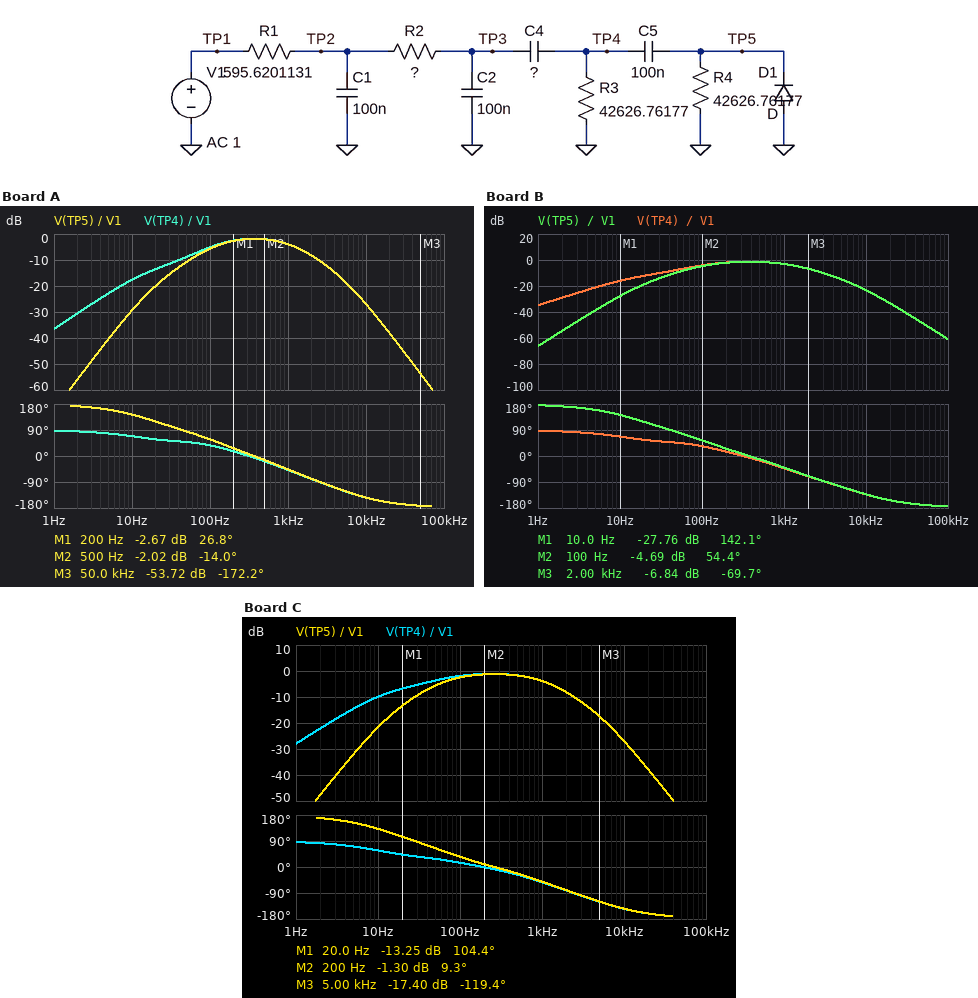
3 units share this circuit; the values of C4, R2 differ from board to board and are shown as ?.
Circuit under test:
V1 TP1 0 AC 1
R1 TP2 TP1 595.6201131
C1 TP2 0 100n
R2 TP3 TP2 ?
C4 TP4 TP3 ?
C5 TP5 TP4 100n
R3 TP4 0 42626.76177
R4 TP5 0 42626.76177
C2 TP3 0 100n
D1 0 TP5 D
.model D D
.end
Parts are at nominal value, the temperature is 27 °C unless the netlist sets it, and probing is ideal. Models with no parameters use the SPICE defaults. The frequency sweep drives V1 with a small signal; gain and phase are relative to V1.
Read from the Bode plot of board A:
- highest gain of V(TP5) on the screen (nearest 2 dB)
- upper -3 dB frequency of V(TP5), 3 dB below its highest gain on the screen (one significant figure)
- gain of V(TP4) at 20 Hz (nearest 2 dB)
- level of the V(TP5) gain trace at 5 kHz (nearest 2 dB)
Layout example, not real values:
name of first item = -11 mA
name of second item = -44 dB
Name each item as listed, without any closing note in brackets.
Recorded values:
highest gain of V(TP5) on the screen = -2 dB
upper -3 dB frequency of V(TP5), 3 dB below its highest gain on the screen = 1 kHz
gain of V(TP4) at 20 Hz = -14 dB
level of the V(TP5) gain trace at 5 kHz = -18 dB
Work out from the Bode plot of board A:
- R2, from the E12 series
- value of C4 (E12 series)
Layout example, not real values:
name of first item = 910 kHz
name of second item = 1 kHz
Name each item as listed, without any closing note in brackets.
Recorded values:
R2, from the E12 series = 820 Ω
value of C4 = 56 nF
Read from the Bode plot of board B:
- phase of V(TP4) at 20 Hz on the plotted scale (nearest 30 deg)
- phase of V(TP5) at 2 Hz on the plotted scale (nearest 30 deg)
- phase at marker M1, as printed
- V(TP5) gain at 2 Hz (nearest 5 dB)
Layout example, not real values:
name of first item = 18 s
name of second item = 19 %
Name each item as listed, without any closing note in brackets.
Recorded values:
phase of V(TP4) at 20 Hz on the plotted scale = 60 deg
phase of V(TP5) at 2 Hz on the plotted scale = 180 deg
phase at marker M1, as printed = 142.1 deg
V(TP5) gain at 2 Hz = -55 dB
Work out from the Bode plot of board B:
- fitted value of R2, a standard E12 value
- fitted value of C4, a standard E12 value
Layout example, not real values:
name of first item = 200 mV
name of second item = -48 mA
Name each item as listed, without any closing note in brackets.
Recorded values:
fitted value of R2, a standard E12 value = 470 Ω
fitted value of C4, a standard E12 value = 68 nF
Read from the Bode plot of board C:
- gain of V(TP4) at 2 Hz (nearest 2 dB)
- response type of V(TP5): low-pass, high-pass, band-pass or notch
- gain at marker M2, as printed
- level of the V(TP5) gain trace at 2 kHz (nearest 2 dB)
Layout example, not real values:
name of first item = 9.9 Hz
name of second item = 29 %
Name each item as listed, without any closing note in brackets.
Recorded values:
gain of V(TP4) at 2 Hz = -22 dB
response type of V(TP5): low-pass, high-pass, band-pass or notch = band-pass
gain at marker M2, as printed = -1.30 dB
level of the V(TP5) gain trace at 2 kHz = -8 dB
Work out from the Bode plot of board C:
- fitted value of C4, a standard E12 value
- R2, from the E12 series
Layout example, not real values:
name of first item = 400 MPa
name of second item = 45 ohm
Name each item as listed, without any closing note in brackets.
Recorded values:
fitted value of C4, a standard E12 value = 150 nF
R2, from the E12 series = 820 Ω
